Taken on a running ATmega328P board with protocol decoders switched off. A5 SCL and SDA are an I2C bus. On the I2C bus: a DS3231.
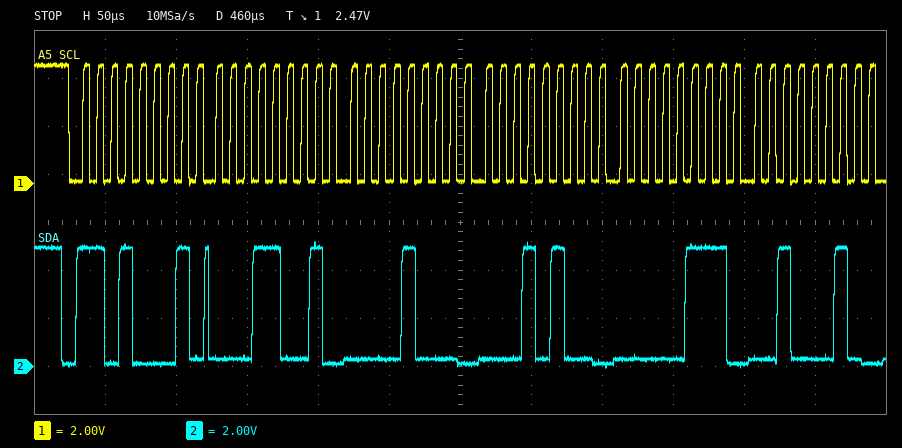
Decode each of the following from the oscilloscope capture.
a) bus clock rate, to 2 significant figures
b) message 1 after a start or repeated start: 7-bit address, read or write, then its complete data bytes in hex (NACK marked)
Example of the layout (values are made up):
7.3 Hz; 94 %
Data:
100 kHz; 0x68 read: 19 08 14 07 22
